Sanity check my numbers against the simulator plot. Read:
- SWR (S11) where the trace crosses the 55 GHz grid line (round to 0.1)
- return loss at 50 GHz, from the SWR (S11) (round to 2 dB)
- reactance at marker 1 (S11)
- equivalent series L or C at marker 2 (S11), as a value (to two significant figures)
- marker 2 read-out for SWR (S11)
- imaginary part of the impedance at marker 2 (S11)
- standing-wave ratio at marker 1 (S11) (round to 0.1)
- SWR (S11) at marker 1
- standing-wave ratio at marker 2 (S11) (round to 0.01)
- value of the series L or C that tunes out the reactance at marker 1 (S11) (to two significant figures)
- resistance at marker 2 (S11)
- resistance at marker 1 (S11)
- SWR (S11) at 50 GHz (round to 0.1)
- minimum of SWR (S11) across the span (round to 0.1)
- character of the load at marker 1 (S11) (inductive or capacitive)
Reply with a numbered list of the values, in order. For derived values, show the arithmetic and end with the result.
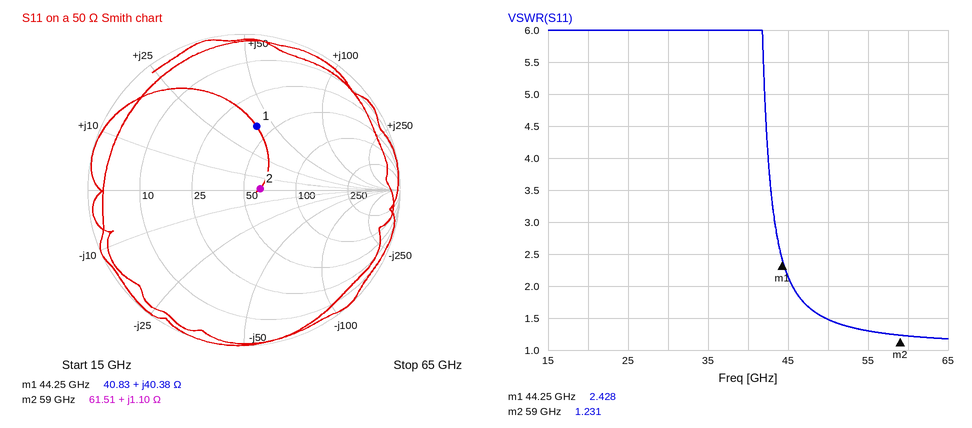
1. 1.3
2. −20 log10((1.5 − 1)/(1.5 + 1)) ≈ 14 dB
3. +40.38 Ω
4. L = 1.1 Ω/(2π × 59 GHz) ≈ 3.0 pH
5. 1.231
6. +1.10 Ω
7. 2.4
8. 2.428
9. 1.23
10. C = 1/(2π × 44.25 GHz × 40.38 Ω) ≈ 89 fF
11. 61.51 Ω
12. 40.83 Ω
13. 1.5
14. 1.2
15. inductive
